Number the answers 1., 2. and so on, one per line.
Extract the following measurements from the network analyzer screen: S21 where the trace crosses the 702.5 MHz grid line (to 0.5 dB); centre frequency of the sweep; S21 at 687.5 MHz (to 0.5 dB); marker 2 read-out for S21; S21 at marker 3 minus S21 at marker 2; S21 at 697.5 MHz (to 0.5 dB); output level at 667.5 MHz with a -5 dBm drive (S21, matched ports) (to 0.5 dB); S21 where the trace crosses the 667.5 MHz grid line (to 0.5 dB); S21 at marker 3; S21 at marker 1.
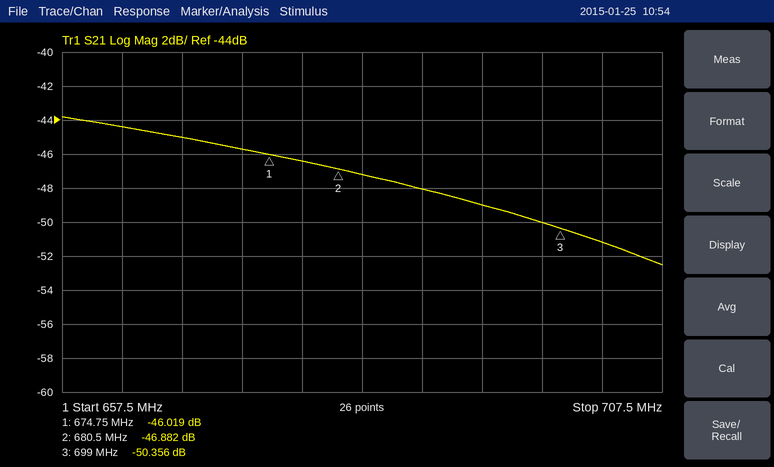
1. -51.0 dB
2. 682.5 MHz
3. -48.0 dB
4. -46.882 dB
5. -3.474 dB
6. -50.0 dB
7. -50.0 dBm
8. -45.0 dB
9. -50.356 dB
10. -46.019 dB
